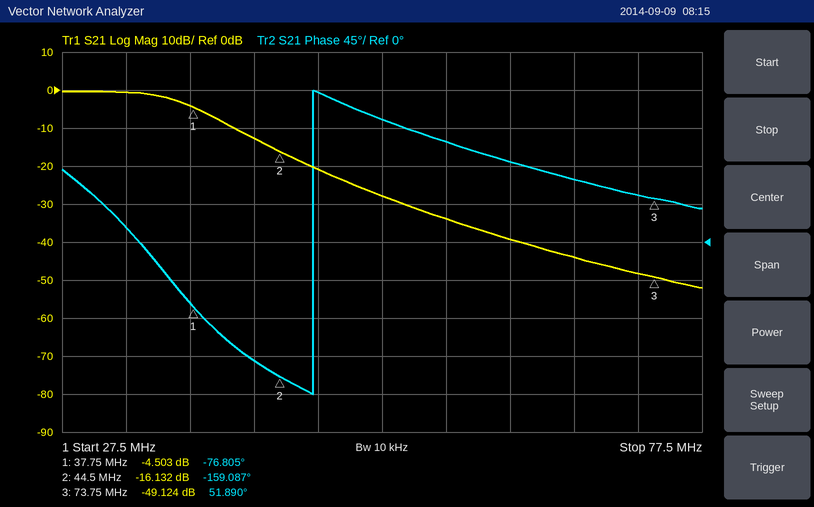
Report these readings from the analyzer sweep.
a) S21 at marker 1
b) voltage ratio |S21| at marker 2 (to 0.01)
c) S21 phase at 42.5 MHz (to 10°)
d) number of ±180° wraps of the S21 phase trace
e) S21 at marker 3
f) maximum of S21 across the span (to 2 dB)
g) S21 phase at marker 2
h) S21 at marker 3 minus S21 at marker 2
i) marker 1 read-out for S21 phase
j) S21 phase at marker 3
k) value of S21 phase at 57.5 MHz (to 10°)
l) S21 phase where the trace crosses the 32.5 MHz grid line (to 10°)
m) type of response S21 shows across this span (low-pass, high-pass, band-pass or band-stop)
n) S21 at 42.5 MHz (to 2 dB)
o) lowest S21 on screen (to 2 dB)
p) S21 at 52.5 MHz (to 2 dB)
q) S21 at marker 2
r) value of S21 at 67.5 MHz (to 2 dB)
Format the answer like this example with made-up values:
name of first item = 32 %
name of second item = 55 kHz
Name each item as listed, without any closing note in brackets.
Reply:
S21 at marker 1 = -4.503 dB
voltage ratio |S21| at marker 2 = 0.16
S21 phase at 42.5 MHz = -140°
number of ±180° wraps of the S21 phase trace = 1
S21 at marker 3 = -49.124 dB
maximum of S21 across the span = 0 dB
S21 phase at marker 2 = -159.087°
S21 at marker 3 minus S21 at marker 2 = -32.992 dB
marker 1 read-out for S21 phase = -76.805°
S21 phase at marker 3 = 51.890°
value of S21 phase at 57.5 MHz = 120°
S21 phase where the trace crosses the 32.5 MHz grid line = 20°
type of response S21 shows across this span = low-pass
S21 at 42.5 MHz = -12 dB
lowest S21 on screen = -52 dB
S21 at 52.5 MHz = -28 dB
S21 at marker 2 = -16.132 dB
value of S21 at 67.5 MHz = -44 dB
